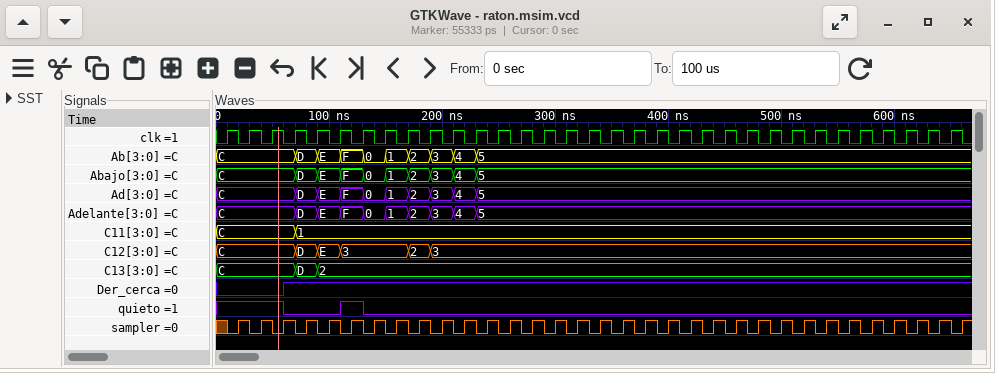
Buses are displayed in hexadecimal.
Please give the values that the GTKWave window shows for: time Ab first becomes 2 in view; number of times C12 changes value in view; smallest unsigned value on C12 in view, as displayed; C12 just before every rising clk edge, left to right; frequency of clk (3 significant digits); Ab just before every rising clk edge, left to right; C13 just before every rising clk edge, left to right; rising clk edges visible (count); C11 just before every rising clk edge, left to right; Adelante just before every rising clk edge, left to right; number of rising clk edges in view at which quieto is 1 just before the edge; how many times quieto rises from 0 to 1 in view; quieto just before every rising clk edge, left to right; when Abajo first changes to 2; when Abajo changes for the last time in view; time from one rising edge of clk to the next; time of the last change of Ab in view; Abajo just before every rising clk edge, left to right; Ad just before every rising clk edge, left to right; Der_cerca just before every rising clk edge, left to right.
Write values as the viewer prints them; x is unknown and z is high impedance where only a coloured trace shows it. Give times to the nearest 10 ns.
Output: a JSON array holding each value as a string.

["170 ns", "5", "2", "C, C, C, C, D, E, 3, 3, 3, 2, 3, 3, 3, 3, 3, 3, 3, 3, 3, 3, 3, 3, 3, 3, 3, 3, 3, 3, 3, 3, 3, 3, 3", "50.0 MHz", "C, C, C, C, D, E, F, 0, 1, 2, 3, 4, 5, 5, 5, 5, 5, 5, 5, 5, 5, 5, 5, 5, 5, 5, 5, 5, 5, 5, 5, 5, 5", "C, C, C, C, D, 2, 2, 2, 2, 2, 2, 2, 2, 2, 2, 2, 2, 2, 2, 2, 2, 2, 2, 2, 2, 2, 2, 2, 2, 2, 2, 2, 2", "33", "C, C, C, C, 1, 1, 1, 1, 1, 1, 1, 1, 1, 1, 1, 1, 1, 1, 1, 1, 1, 1, 1, 1, 1, 1, 1, 1, 1, 1, 1, 1, 1", "C, C, C, C, D, E, F, 0, 1, 2, 3, 4, 5, 5, 5, 5, 5, 5, 5, 5, 5, 5, 5, 5, 5, 5, 5, 5, 5, 5, 5, 5, 5", "4", "1", "1 1 1 0 0 0 1 0 0 0 0 0 0 0 0 0 0 0 0 0 0 0 0 0 0 0 0 0 0 0 0 0 0", "170 ns", "230 ns", "20 ns", "230 ns", "C, C, C, C, D, E, F, 0, 1, 2, 3, 4, 5, 5, 5, 5, 5, 5, 5, 5, 5, 5, 5, 5, 5, 5, 5, 5, 5, 5, 5, 5, 5", "C, C, C, C, D, E, F, 0, 1, 2, 3, 4, 5, 5, 5, 5, 5, 5, 5, 5, 5, 5, 5, 5, 5, 5, 5, 5, 5, 5, 5, 5, 5", "0 0 0 1 1 1 1 1 1 1 1 1 1 1 1 1 1 1 1 1 1 1 1 1 1 1 1 1 1 1 1 1 1"]
